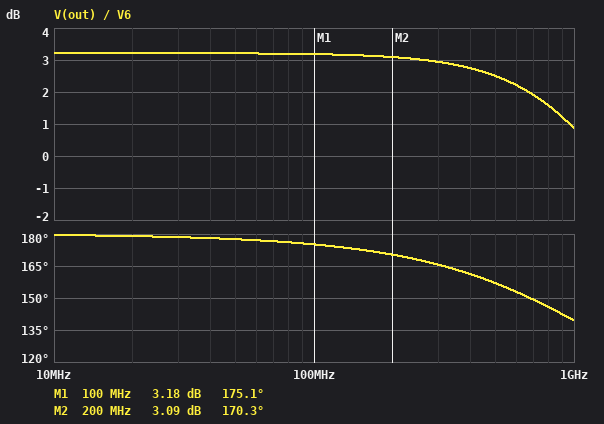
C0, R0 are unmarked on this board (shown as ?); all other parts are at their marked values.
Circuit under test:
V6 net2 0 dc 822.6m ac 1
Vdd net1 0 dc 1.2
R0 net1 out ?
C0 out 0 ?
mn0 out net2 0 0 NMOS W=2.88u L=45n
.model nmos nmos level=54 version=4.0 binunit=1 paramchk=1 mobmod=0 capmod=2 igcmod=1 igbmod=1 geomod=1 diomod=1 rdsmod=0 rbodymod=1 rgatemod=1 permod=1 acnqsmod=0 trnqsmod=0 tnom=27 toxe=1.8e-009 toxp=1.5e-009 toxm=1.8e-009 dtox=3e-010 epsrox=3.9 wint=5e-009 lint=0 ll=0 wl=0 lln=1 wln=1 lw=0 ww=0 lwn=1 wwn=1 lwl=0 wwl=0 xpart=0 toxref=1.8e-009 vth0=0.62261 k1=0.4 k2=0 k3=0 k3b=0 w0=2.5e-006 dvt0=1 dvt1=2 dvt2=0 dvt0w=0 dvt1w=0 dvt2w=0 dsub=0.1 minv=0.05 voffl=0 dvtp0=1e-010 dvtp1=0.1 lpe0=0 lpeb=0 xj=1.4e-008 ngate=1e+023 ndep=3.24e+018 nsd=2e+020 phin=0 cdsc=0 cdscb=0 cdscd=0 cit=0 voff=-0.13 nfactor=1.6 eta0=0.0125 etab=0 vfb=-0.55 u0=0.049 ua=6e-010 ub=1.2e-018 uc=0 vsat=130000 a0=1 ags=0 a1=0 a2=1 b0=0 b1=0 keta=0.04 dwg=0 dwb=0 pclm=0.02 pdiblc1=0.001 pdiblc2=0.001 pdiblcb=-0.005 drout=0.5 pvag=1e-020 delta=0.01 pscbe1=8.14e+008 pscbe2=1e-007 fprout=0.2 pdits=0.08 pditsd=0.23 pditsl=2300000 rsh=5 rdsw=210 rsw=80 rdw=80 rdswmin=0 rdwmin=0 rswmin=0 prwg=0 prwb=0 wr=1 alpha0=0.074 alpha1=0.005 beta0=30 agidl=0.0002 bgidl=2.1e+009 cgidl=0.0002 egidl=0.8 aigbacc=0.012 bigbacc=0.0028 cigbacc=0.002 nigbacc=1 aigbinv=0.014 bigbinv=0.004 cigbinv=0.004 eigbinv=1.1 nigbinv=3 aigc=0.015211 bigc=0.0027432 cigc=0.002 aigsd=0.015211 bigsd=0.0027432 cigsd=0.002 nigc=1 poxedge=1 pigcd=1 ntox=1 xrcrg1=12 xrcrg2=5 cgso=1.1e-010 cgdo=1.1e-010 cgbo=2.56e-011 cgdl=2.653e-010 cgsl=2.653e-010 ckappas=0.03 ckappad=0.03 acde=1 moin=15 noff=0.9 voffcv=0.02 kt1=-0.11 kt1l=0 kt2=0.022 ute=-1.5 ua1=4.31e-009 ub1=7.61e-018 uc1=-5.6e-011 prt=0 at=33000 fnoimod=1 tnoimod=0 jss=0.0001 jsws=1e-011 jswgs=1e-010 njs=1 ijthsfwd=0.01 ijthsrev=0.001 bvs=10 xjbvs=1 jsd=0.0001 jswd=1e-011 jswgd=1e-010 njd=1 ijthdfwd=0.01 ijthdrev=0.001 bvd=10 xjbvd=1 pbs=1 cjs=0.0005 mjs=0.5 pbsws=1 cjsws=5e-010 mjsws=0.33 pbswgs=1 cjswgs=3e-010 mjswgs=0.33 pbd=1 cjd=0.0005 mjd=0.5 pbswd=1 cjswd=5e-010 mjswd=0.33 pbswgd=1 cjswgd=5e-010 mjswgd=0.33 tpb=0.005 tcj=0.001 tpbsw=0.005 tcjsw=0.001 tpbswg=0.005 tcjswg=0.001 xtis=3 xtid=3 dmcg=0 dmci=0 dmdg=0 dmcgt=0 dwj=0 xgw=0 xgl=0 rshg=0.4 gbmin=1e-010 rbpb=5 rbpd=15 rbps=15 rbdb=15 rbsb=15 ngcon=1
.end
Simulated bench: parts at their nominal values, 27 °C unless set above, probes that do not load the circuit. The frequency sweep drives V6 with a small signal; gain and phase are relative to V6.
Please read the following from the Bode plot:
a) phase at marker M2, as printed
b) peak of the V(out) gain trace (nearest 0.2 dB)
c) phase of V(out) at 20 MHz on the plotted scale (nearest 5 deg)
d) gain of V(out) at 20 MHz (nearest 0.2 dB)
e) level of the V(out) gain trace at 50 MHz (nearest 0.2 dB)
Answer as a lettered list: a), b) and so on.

a) 170.3 deg
b) 3.2 dB
c) 180 deg
d) 3.2 dB
e) 3.2 dB
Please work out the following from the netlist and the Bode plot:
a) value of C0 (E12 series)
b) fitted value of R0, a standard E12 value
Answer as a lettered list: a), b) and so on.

a) 270 fF
b) 560 Ω
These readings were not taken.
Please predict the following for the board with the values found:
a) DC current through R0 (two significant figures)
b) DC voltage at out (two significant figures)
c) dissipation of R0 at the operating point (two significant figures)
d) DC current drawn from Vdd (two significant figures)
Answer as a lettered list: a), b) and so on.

a) 570 µA
b) 880 mV
c) 180 µW
d) 570 µA
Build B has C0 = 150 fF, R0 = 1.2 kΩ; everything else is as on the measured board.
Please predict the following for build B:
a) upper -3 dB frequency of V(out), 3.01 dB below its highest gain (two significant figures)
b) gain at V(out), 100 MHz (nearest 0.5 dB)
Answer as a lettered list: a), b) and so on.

a) 1.1 GHz
b) 8.5 dB
